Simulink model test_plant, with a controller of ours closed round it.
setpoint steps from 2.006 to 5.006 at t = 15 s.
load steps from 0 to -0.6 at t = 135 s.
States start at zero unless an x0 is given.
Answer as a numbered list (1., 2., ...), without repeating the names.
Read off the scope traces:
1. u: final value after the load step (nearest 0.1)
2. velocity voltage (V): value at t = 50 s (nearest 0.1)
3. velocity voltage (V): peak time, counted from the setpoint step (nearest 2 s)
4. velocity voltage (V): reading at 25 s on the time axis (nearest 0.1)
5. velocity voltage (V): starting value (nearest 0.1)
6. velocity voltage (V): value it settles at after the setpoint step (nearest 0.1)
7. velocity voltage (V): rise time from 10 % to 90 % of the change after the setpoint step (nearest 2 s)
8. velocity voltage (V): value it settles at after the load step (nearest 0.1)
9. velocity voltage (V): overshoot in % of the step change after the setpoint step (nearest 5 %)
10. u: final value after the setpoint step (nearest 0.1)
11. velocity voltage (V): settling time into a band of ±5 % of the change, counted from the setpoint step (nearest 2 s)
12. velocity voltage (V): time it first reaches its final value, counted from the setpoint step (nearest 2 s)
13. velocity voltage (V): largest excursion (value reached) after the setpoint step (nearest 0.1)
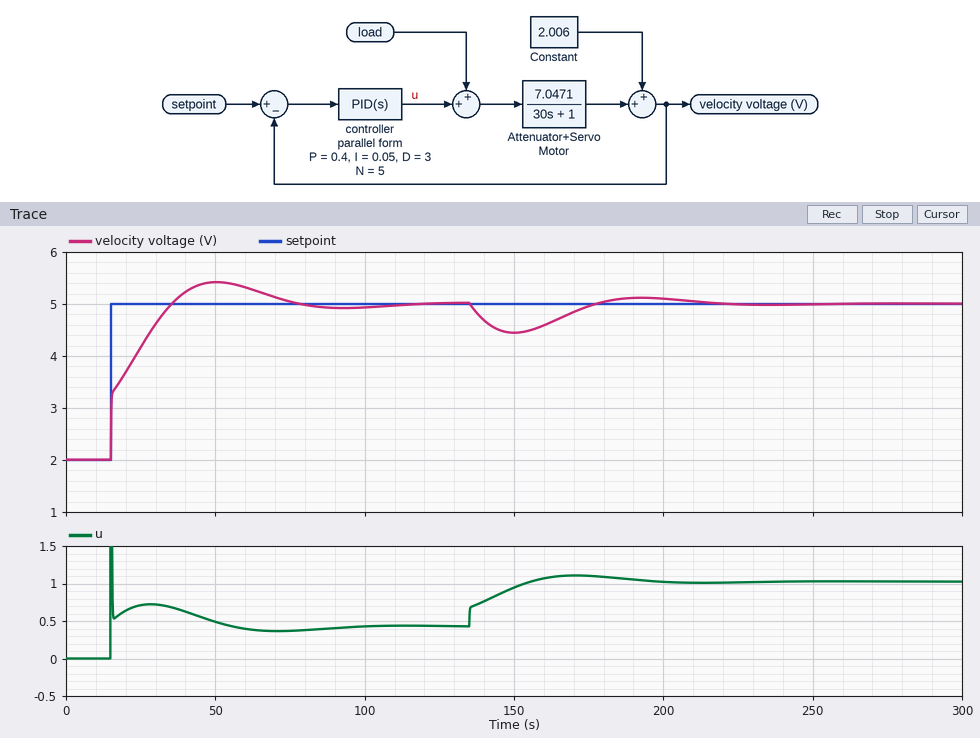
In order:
1. 1.0
2. 5.4
3. 36 s
4. 4.2
5. 2.0
6. 5.0
7. 16 s
8. 5.0
9. 15 %
10. 0.4
11. 54 s
12. 20 s
13. 5.4
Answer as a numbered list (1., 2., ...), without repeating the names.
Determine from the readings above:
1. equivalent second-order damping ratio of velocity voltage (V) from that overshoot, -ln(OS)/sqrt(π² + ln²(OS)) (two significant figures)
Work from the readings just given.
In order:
1. 0.52
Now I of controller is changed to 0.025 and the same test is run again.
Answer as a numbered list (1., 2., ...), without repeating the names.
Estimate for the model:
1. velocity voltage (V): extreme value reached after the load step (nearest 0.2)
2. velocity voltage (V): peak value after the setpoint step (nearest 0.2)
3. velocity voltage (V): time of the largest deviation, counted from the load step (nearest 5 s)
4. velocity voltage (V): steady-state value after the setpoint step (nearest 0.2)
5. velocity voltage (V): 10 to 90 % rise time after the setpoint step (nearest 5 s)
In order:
1. 4.4
2. 5.2
3. 20 s
4. 5.0
5. 25 s
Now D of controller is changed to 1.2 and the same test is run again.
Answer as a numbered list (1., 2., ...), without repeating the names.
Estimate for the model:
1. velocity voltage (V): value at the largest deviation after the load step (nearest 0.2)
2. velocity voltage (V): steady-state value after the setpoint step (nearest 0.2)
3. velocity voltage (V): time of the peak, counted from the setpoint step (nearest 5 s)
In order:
1. 4.4
2. 5.0
3. 30 s
